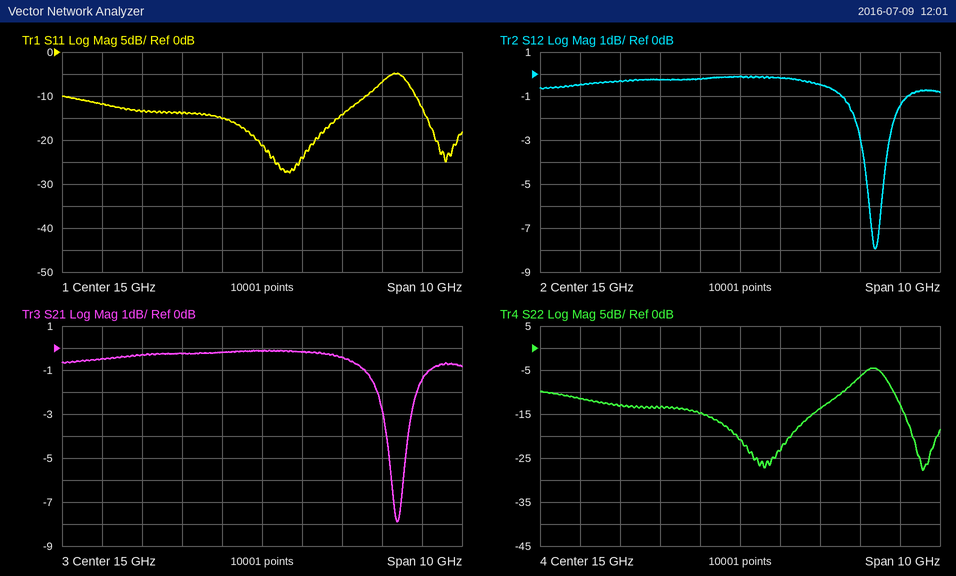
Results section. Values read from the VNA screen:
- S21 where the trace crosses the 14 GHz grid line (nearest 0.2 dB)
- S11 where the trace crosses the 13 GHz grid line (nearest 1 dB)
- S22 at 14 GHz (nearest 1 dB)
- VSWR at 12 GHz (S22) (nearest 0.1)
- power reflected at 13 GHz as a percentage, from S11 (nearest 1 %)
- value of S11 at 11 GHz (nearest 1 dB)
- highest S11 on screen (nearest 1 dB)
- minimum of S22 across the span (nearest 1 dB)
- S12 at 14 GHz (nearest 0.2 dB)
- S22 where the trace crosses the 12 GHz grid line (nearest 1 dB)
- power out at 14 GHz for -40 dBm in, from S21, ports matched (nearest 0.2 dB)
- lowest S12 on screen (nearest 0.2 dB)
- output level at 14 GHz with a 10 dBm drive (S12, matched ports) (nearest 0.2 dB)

-0.2 dB
-14 dB
-15 dB
1.6
4 %
-12 dB
-5 dB
-28 dB
-0.2 dB
-13 dB
-40.2 dBm
-8.0 dB
9.8 dBm
